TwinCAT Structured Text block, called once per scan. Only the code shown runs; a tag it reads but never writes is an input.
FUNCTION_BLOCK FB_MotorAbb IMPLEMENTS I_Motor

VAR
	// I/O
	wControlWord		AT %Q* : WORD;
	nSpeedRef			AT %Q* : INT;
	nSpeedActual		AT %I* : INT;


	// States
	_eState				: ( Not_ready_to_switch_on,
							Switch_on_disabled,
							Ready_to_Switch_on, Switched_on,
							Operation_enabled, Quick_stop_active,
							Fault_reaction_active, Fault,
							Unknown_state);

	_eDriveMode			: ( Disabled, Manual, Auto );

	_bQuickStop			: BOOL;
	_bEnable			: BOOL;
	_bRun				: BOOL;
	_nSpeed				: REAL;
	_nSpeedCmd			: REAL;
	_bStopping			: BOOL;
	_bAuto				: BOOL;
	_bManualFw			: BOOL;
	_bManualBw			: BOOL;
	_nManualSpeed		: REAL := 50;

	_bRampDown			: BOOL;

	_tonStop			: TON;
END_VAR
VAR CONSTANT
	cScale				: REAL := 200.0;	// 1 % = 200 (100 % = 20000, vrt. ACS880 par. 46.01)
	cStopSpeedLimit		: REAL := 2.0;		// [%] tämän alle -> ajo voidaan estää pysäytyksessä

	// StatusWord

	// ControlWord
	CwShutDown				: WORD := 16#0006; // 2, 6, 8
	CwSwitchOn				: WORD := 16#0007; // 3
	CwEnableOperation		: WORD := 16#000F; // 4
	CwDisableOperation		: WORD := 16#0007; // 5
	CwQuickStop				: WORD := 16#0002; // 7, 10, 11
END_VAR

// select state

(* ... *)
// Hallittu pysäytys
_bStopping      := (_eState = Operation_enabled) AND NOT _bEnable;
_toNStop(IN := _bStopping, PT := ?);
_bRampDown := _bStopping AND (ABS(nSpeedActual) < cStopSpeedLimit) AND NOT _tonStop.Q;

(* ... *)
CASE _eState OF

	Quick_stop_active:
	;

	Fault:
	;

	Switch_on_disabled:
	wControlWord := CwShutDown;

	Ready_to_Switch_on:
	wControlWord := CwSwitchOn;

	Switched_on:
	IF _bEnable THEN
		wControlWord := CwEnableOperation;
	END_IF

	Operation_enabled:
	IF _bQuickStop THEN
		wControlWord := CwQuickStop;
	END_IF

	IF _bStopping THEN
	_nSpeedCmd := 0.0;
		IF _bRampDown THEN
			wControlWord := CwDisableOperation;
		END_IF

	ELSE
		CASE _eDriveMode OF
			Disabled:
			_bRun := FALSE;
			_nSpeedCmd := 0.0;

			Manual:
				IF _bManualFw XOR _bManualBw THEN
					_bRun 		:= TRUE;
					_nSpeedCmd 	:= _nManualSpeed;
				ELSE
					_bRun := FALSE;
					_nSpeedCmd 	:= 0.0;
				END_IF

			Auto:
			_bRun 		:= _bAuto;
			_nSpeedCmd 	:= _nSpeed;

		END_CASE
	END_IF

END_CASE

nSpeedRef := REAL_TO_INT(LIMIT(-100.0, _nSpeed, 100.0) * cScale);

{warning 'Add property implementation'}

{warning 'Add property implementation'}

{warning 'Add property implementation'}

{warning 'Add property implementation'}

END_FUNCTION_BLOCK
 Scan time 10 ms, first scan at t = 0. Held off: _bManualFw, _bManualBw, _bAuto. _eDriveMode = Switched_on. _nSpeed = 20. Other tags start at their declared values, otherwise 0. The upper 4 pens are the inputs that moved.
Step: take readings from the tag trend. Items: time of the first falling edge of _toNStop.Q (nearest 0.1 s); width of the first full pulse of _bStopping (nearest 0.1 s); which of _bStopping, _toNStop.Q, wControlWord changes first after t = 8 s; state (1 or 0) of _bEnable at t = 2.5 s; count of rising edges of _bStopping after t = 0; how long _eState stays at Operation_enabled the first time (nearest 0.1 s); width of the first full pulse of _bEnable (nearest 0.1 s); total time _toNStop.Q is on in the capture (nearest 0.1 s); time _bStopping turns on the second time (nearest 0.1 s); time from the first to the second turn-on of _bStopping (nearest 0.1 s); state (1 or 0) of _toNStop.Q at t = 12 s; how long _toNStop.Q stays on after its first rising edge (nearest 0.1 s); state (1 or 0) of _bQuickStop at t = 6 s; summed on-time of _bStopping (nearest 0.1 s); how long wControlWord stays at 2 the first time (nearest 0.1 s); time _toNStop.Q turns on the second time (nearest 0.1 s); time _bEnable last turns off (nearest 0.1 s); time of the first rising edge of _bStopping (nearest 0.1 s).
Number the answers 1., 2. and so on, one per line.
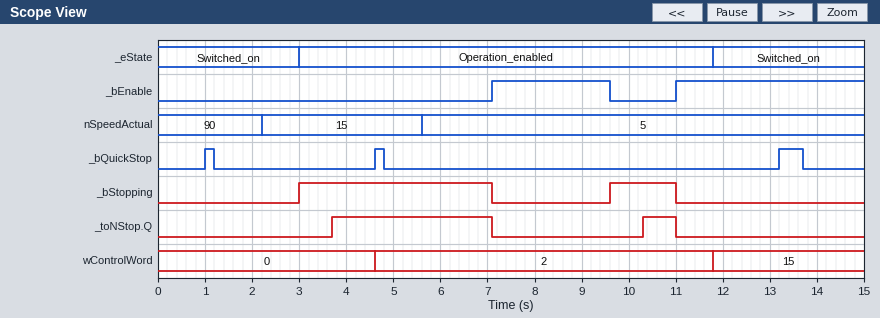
1. 7.1 s
2. 4.1 s
3. _bStopping
4. 0
5. 2
6. 8.8 s
7. 2.5 s
8. 4.1 s
9. 9.6 s
10. 6.6 s
11. 0
12. 3.4 s
13. 0
14. 5.5 s
15. 7.2 s
16. 10.3 s
17. 9.6 s
18. 3.0 s
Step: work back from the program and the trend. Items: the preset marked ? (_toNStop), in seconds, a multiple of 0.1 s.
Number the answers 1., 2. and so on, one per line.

1. 0.7 s
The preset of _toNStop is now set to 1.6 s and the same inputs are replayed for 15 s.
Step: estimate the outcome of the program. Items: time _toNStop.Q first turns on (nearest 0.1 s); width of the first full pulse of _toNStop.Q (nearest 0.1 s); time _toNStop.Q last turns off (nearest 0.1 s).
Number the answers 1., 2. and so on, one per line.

1. 4.6 s
2. 2.5 s
3. 7.1 s
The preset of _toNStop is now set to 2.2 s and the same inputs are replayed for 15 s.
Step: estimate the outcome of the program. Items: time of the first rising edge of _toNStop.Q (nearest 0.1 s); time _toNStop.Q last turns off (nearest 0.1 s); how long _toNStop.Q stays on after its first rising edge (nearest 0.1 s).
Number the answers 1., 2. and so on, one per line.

1. 5.2 s
2. 7.1 s
3. 1.9 s
